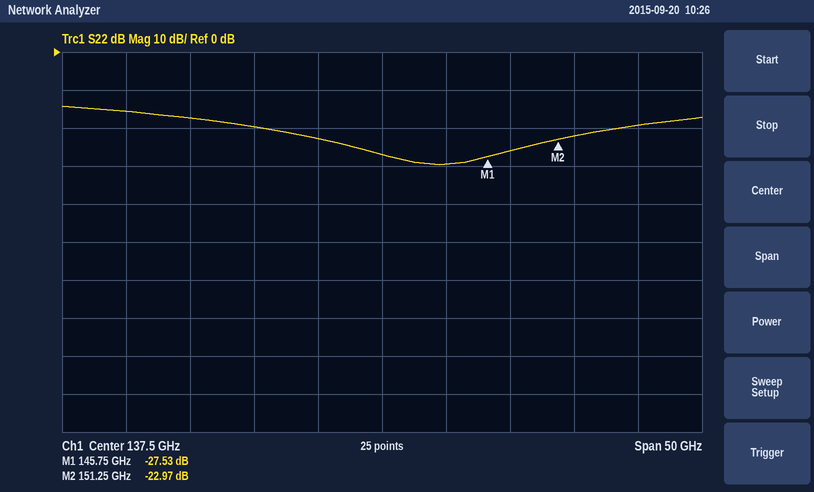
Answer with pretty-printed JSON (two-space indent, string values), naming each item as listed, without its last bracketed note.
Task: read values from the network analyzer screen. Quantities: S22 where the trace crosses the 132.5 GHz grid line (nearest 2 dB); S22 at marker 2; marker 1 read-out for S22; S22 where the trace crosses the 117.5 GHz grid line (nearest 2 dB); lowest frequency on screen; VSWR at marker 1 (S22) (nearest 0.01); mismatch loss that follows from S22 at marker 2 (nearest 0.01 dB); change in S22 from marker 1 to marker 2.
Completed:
{
  "S22 where the trace crosses the 132.5 GHz grid line": "-22 dB",
  "S22 at marker 2": "-22.97 dB",
  "marker 1 read-out for S22": "-27.53 dB",
  "S22 where the trace crosses the 117.5 GHz grid line": "-16 dB",
  "lowest frequency on screen": "112.5 GHz",
  "VSWR at marker 1 (S22)": "1.09",
  "mismatch loss that follows from S22 at marker 2": "0.02 dB",
  "change in S22 from marker 1 to marker 2": "4.56 dB"
}
